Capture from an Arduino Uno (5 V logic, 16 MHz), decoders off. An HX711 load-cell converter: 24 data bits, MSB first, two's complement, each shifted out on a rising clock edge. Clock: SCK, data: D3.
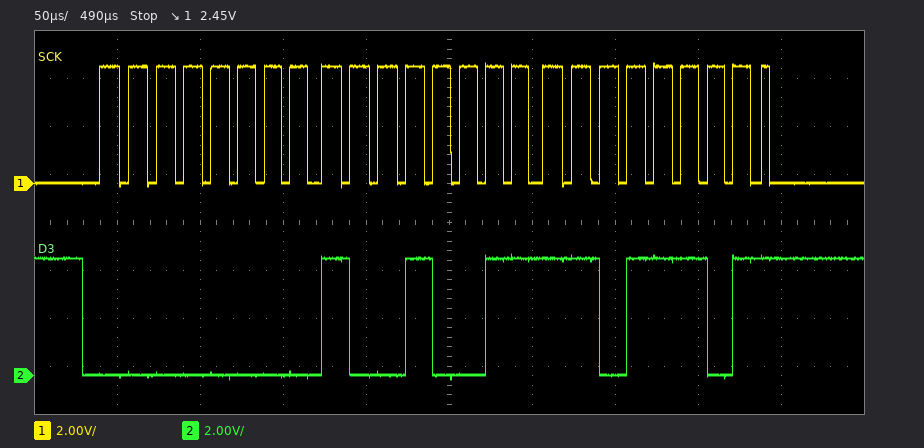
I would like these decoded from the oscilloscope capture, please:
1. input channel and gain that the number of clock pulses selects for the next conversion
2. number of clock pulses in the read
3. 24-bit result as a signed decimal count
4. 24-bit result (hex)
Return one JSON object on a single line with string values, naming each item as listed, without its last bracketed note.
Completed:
{"input channel and gain that the number of clock pulses selects for the next conversion": "channel A, gain 128", "number of clock pulses in the read": "25", "24-bit result as a signed decimal count": "37853", "24-bit result": "0x0093DD"}
